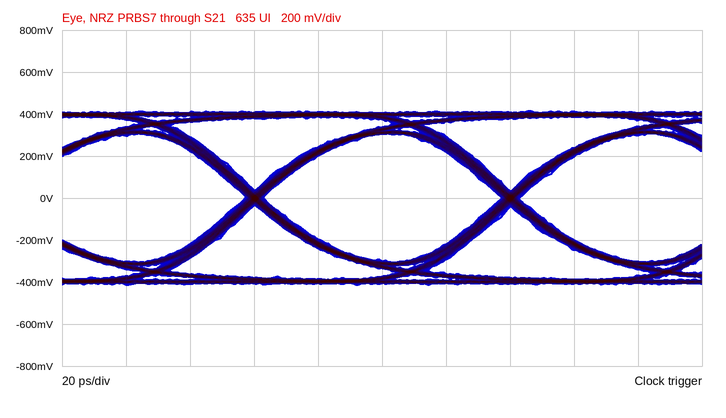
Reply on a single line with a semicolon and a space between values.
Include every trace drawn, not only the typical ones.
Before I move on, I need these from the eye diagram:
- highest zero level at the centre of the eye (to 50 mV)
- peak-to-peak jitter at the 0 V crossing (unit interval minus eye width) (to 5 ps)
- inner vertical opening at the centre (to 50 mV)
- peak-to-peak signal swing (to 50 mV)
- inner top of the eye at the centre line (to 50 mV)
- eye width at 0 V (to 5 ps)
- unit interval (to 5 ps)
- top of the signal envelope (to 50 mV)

-300 mV; 5 ps; 600 mV; 850 mV; 300 mV; 75 ps; 80 ps; 400 mV
